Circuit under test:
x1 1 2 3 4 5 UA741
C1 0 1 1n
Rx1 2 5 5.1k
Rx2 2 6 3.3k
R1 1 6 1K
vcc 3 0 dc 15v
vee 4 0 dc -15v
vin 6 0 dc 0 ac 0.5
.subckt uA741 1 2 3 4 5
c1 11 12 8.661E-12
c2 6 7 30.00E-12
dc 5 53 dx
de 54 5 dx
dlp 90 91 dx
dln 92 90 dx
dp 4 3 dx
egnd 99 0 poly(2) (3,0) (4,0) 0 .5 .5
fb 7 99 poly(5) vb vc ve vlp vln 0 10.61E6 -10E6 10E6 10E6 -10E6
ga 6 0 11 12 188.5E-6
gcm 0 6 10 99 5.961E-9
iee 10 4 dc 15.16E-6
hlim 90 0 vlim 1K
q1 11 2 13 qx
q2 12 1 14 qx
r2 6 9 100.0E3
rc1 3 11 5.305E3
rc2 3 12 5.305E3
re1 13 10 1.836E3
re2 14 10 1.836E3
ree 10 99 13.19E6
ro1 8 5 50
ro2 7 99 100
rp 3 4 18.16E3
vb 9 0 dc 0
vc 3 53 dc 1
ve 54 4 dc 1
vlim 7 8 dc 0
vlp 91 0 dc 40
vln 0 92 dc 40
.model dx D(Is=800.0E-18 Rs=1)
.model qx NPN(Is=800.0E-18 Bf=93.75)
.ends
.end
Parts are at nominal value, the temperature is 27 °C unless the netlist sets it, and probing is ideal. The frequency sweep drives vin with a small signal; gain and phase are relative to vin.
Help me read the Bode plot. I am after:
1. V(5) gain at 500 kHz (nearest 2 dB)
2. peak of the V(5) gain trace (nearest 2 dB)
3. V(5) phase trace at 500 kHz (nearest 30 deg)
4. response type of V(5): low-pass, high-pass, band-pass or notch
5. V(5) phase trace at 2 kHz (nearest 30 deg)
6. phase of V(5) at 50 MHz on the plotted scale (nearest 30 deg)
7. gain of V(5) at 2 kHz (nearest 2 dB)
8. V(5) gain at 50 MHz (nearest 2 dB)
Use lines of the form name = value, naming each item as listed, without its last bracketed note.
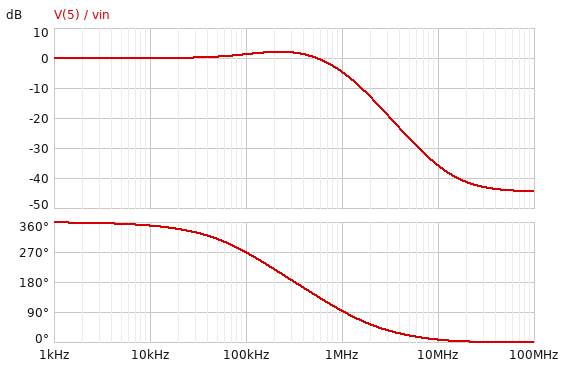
V(5) gain at 500 kHz = 0 dB
peak of the V(5) gain trace = 2 dB
V(5) phase trace at 500 kHz = 150 deg
response type of V(5): low-pass, high-pass, band-pass or notch = low-pass
V(5) phase trace at 2 kHz = 360 deg
phase of V(5) at 50 MHz on the plotted scale = 0 deg
gain of V(5) at 2 kHz = 0 dB
V(5) gain at 50 MHz = -44 dB
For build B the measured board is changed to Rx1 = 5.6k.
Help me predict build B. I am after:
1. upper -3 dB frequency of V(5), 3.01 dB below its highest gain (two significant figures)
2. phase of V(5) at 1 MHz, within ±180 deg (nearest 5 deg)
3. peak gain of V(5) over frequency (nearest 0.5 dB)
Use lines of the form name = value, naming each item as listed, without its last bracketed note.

upper -3 dB frequency of V(5), 3.01 dB below its highest gain = 620 kHz
phase of V(5) at 1 MHz, within ±180 deg = 90 deg
peak gain of V(5) over frequency = 2.5 dB
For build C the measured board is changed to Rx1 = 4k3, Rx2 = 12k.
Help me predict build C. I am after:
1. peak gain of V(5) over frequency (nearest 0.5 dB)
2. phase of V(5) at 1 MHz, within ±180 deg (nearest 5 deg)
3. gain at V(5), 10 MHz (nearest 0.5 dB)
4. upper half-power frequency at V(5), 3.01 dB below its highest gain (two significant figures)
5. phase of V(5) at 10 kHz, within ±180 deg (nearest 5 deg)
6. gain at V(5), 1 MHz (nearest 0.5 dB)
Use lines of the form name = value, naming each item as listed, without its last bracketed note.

peak gain of V(5) over frequency = 0 dB
phase of V(5) at 1 MHz, within ±180 deg = 130 deg
gain at V(5), 10 MHz = -42.5 dB
upper half-power frequency at V(5), 3.01 dB below its highest gain = 180 kHz
phase of V(5) at 10 kHz, within ±180 deg = -5 deg
gain at V(5), 1 MHz = -11.0 dB
